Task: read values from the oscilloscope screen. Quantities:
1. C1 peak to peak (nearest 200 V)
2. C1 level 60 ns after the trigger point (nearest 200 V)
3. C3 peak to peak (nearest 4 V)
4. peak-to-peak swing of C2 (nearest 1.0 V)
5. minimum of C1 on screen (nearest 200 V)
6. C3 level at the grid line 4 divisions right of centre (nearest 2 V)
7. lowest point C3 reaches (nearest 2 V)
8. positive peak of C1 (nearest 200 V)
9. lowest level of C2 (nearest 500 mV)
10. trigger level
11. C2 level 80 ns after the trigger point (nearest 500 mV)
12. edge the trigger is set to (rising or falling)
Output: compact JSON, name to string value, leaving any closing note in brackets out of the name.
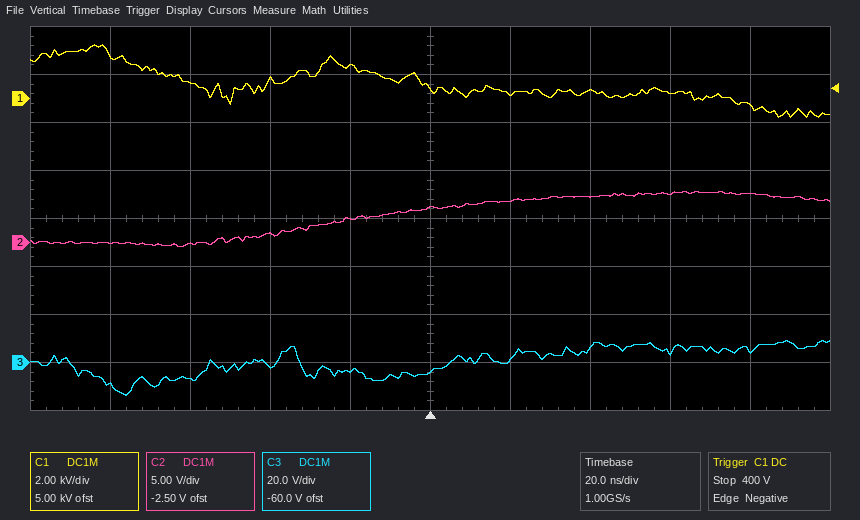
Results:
{"C1 peak to peak": "3.0 kV", "C1 level 60 ns after the trigger point": "200 V", "C3 peak to peak": "24 V", "peak-to-peak swing of C2": "6.0 V", "minimum of C1 on screen": "-800 V", "C3 level at the grid line 4 divisions right of centre": "6 V", "lowest point C3 reaches": "-14 V", "positive peak of C1": "2.2 kV", "lowest level of C2": "-500 mV", "trigger level": "400 V", "C2 level 80 ns after the trigger point": "5.0 V", "edge the trigger is set to": "falling"}
